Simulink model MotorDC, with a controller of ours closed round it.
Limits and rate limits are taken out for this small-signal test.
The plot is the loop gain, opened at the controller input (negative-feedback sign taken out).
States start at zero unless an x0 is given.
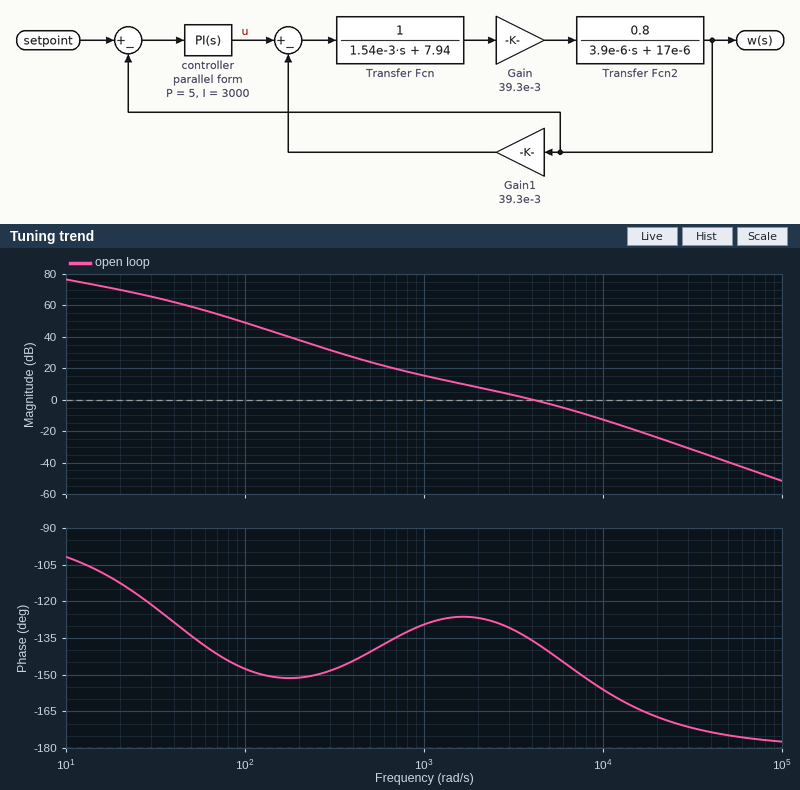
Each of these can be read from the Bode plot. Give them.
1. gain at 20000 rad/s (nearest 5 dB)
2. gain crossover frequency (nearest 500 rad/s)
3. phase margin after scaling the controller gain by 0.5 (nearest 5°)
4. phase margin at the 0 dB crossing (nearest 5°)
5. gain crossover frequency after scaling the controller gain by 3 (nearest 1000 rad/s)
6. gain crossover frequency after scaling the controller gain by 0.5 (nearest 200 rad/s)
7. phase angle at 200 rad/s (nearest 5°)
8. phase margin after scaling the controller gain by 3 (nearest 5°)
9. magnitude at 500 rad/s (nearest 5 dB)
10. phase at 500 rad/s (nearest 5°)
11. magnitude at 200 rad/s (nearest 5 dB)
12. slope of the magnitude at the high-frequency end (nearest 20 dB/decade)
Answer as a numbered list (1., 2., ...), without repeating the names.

1. -25 dB
2. 4000 rad/s
3. 50°
4. 45°
5. 8000 rad/s
6. 2400 rad/s
7. -150°
8. 30°
9. 25 dB
10. -140°
11. 40 dB
12. -40 dB/decade
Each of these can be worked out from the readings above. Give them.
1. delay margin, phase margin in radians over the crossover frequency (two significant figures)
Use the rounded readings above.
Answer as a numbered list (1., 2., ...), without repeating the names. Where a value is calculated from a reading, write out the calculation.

1. 45 × π / 180 / 4000 = 0.00020 s
